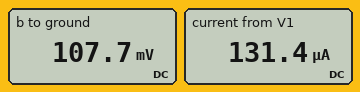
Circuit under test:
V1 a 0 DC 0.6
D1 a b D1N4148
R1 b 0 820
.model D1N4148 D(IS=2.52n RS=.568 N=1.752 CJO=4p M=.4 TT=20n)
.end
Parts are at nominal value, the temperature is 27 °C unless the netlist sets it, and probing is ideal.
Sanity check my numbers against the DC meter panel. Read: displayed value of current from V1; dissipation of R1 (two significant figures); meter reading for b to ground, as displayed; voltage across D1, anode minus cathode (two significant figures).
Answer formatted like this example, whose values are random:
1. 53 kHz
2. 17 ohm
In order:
1. 131.4 µA
2. 14 µW
3. 107.7 mV
4. 490 mV
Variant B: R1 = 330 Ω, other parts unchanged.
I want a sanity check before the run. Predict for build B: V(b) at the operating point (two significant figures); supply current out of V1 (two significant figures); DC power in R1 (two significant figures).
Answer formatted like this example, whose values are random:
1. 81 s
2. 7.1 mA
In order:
1. 80 mV
2. 240 µA
3. 19 µW
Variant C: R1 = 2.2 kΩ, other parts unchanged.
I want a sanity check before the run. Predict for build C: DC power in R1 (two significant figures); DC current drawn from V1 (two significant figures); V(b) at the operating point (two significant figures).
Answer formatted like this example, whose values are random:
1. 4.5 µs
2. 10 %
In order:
1. 9.0 µW
2. 64 µA
3. 140 mV
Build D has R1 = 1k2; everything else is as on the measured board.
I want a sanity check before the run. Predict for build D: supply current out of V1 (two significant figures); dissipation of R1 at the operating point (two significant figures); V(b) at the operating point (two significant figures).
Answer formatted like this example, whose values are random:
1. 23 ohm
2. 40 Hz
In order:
1. 100 µA
2. 12 µW
3. 120 mV
